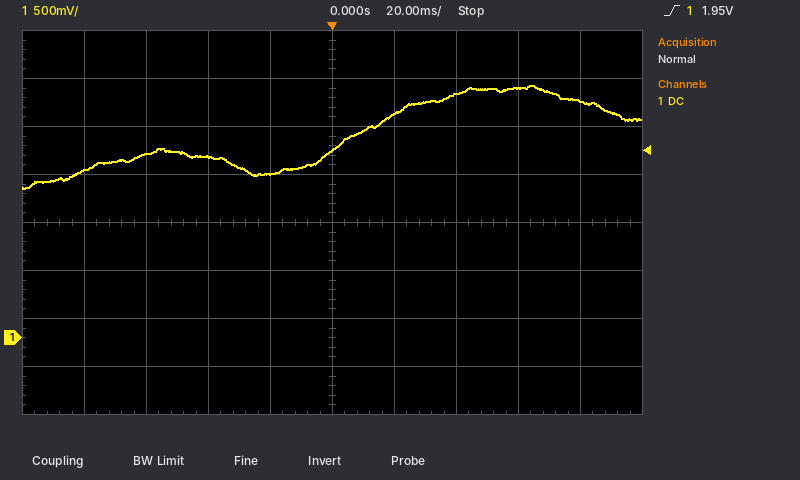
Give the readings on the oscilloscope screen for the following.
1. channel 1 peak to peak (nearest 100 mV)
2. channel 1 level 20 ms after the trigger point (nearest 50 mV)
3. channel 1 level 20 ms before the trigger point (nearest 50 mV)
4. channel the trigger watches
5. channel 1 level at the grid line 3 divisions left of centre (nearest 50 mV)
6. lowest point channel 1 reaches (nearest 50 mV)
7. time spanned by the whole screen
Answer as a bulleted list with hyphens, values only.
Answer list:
- 1.10 V
- 2.35 V
- 1.70 V
- channel 1
- 1.90 V
- 1.55 V
- 200 ms
